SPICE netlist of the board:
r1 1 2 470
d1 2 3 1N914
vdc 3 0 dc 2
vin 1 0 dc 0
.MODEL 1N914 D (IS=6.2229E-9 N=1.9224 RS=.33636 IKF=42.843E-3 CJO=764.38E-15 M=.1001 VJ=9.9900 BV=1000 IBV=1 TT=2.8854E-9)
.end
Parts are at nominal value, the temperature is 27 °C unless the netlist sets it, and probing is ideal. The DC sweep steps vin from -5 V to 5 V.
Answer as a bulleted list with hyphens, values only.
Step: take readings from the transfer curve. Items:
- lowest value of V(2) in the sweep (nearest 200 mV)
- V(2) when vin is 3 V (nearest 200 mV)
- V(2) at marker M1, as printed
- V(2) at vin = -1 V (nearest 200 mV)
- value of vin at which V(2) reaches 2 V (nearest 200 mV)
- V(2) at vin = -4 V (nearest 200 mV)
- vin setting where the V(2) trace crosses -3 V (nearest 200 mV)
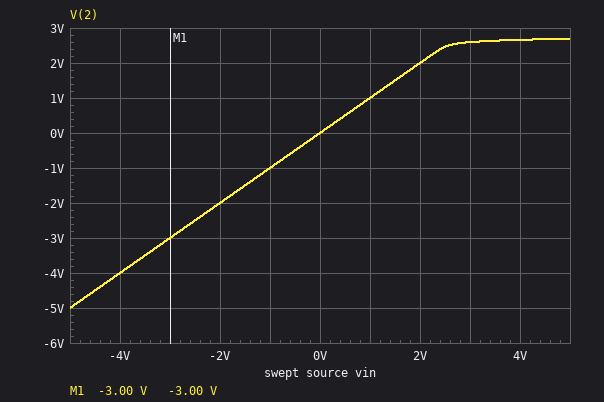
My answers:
- -5.0 V
- 2.6 V
- -3.00 V
- -1.0 V
- 2.0 V
- -4.0 V
- -3.0 V
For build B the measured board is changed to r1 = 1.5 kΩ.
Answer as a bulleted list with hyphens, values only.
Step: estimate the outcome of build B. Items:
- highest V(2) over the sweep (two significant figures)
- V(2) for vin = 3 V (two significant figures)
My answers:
- 2.6 V
- 2.5 V
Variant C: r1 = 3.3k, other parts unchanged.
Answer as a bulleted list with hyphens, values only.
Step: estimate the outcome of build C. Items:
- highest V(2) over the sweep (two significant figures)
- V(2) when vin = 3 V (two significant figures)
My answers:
- 2.6 V
- 2.5 V
